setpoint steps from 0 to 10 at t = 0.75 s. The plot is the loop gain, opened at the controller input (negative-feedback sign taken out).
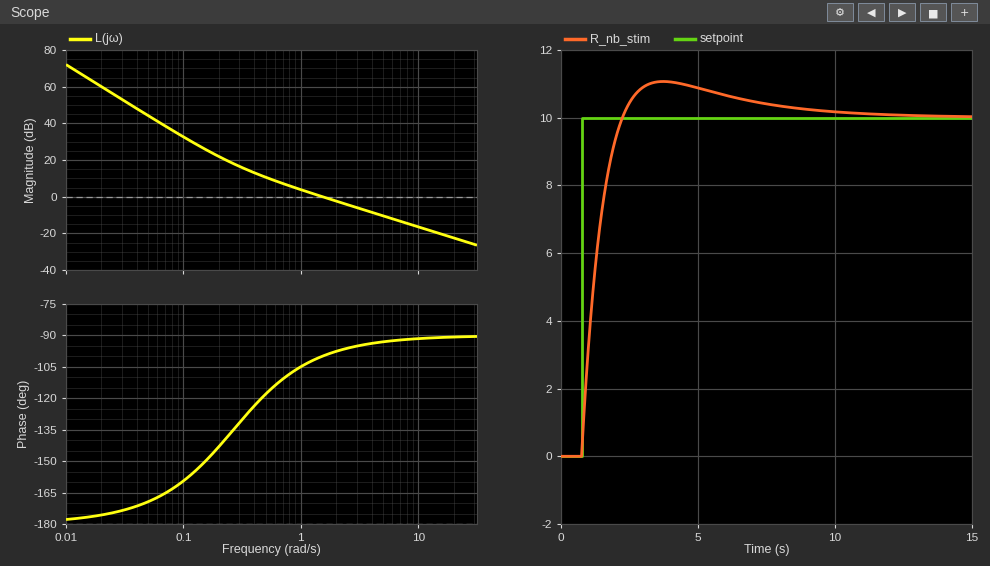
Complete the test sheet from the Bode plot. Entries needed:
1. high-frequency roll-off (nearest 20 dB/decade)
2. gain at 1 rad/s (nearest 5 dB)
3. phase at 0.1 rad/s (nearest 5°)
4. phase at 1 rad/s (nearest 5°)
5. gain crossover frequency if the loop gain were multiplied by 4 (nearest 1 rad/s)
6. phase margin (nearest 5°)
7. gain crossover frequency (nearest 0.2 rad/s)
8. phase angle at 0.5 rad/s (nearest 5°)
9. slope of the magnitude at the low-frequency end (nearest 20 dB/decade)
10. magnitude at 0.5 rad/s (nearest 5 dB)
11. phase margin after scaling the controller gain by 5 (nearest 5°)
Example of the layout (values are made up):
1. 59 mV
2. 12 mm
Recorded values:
1. -20 dB/decade
2. 5 dB
3. -160°
4. -105°
5. 6 rad/s
6. 80°
7. 1.6 rad/s
8. -120°
9. -40 dB/decade
10. 10 dB
11. 90°
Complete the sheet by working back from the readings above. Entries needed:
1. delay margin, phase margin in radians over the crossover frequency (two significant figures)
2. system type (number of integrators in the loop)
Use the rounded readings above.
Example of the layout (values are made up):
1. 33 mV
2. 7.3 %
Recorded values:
1. 0.87 s
2. 2
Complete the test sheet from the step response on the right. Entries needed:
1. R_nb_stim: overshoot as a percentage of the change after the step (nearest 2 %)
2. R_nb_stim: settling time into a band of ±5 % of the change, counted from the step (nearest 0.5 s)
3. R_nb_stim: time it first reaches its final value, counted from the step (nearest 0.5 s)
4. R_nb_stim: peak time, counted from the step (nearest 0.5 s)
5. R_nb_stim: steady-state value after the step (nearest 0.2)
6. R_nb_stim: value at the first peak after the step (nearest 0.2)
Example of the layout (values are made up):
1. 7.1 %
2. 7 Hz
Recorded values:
1. 10 %
2. 6.0 s
3. 1.5 s
4. 3.0 s
5. 10.0
6. 11.0
